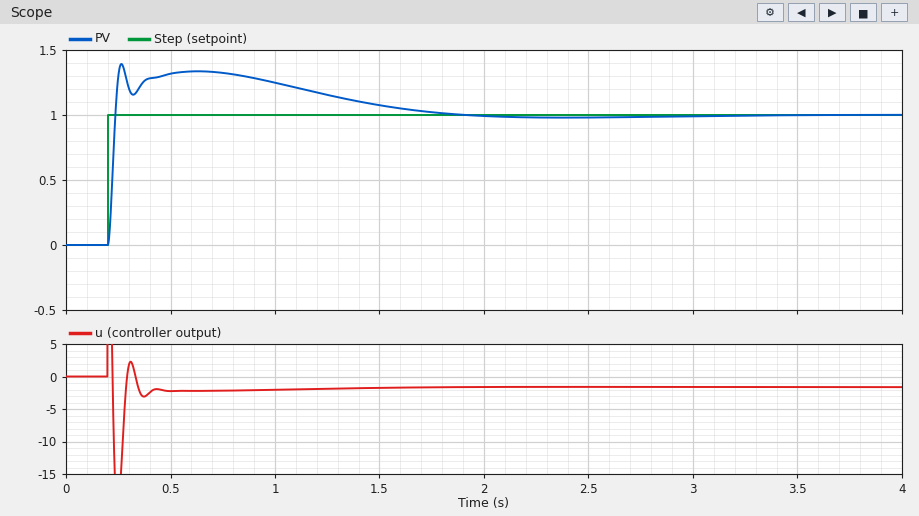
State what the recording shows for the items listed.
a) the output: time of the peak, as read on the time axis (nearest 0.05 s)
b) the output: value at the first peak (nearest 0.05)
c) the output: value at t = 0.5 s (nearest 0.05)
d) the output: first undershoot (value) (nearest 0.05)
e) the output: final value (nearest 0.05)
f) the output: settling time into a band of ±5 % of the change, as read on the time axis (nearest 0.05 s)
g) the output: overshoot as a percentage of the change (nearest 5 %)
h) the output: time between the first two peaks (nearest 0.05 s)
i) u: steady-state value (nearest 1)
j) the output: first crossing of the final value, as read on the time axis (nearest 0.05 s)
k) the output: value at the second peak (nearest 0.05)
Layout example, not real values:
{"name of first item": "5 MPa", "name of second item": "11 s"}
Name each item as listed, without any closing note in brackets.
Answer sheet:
{"the output: time of the peak, as read on the time axis": "0.25 s", "the output: value at the first peak": "1.40", "the output: value at t = 0.5 s": "1.30", "the output: first undershoot (value)": "1.15", "the output: final value": "1.00", "the output: settling time into a band of ±5 % of the change, as read on the time axis": "1.60 s", "the output: overshoot as a percentage of the change": "40 %", "the output: time between the first two peaks": "0.35 s", "u: steady-state value": "-2", "the output: first crossing of the final value, as read on the time axis": "0.25 s", "the output: value at the second peak": "1.35"}
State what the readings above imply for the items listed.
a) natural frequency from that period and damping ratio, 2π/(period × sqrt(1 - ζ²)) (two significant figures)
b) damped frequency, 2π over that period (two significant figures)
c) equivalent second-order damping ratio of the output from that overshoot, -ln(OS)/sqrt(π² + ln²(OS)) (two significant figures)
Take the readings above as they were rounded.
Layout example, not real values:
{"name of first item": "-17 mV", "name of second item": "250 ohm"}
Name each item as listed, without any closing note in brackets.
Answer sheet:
{"natural frequency from that period and damping ratio, 2π/(period × sqrt(1 - ζ²))": "19 rad/s", "damped frequency, 2π over that period": "18 rad/s", "equivalent second-order damping ratio of the output from that overshoot, -ln(OS)/sqrt(π² + ln²(OS))": "0.28"}
